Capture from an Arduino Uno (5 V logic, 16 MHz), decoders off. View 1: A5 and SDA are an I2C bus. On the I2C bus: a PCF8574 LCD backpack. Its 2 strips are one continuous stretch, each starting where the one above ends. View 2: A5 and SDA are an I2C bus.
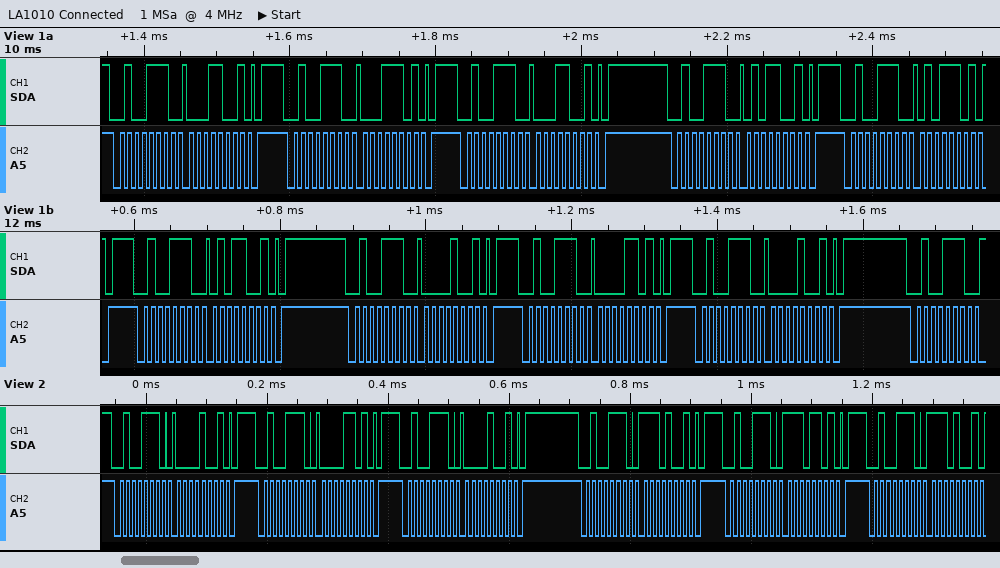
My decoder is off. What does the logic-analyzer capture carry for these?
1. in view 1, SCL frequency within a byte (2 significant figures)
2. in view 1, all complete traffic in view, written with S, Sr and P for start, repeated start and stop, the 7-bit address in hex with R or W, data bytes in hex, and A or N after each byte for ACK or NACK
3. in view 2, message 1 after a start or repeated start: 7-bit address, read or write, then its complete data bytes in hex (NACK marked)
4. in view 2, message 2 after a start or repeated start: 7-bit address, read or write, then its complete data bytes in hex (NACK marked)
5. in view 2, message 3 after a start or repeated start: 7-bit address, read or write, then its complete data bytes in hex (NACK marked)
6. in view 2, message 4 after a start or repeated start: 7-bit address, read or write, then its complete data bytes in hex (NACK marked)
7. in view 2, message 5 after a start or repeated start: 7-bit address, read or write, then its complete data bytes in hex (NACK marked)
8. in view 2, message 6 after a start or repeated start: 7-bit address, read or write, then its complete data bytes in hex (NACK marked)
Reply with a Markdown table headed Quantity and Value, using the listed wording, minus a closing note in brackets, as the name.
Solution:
| Quantity | Value |
|---|---|
| in view 1, SCL frequency within a byte | 100 kHz |
| in view 1, all complete traffic in view, written with S, Sr and P for start, repeated start and stop, the 7-bit address in hex with R or W, data bytes in hex, and A or N after each byte for ACK or NACK | S 27W A 19 A P S 27W A 1D A P S 27W A 19 A P S 27W A 59 A P S 27W A 5D A P S 27W A 59 A P S 27W A 09 A P S 27W A 0D A P S 27W A 09 A P S 27W A |
| in view 2, message 1 after a start or repeated start: 7-bit address, read or write, then its complete data bytes in hex | 0x27 write: 09 |
| in view 2, message 2 after a start or repeated start: 7-bit address, read or write, then its complete data bytes in hex | 0x27 write: 0D |
| in view 2, message 3 after a start or repeated start: 7-bit address, read or write, then its complete data bytes in hex | 0x27 write: 09 |
| in view 2, message 4 after a start or repeated start: 7-bit address, read or write, then its complete data bytes in hex | 0x27 write: E9 |
| in view 2, message 5 after a start or repeated start: 7-bit address, read or write, then its complete data bytes in hex | 0x27 write: ED |
| in view 2, message 6 after a start or repeated start: 7-bit address, read or write, then its complete data bytes in hex | 0x27 write: E9 |
